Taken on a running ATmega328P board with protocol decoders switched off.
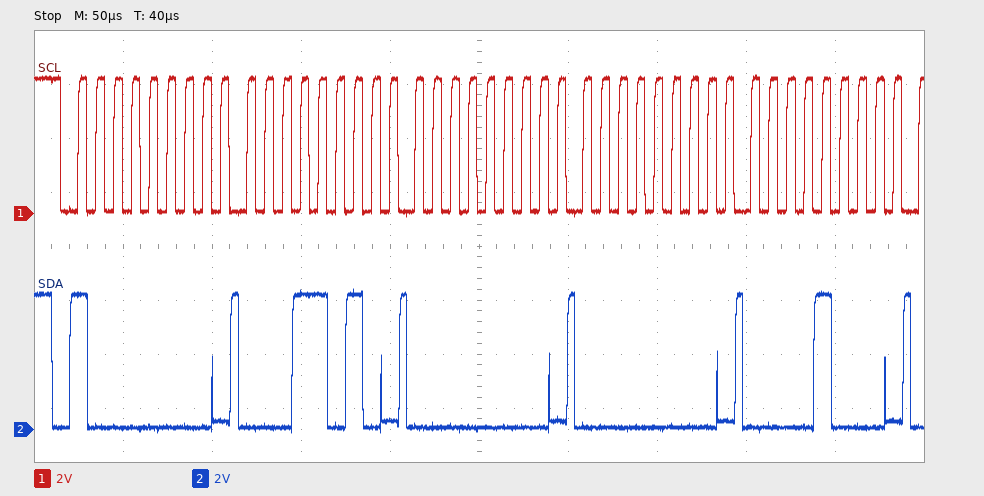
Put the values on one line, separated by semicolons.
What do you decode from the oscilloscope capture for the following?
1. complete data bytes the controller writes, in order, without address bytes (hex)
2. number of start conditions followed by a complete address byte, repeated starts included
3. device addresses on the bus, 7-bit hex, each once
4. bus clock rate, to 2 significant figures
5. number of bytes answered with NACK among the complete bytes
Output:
1A 00 00 08; 1; 0x40; 100 kHz; 0
